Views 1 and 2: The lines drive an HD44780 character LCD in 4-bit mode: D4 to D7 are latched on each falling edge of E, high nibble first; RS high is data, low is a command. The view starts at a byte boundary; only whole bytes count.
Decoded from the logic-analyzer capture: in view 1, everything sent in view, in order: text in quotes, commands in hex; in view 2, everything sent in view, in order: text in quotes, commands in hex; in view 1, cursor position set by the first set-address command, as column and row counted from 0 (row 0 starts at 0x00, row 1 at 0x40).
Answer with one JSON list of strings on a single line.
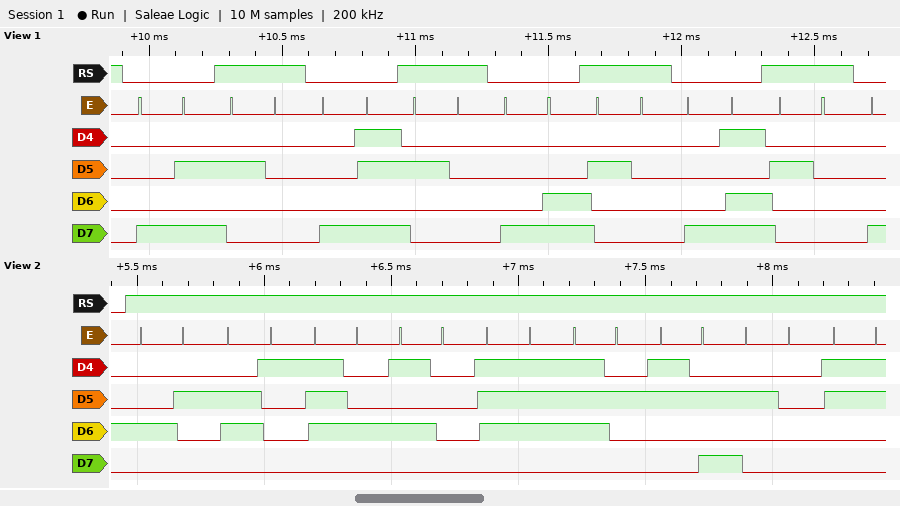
["0x8A \" \" 0x8B \" \" 0x8C \" \" 0x8D \" \"", "\"BatPwr: 3\"", "column 10, row 0"]
